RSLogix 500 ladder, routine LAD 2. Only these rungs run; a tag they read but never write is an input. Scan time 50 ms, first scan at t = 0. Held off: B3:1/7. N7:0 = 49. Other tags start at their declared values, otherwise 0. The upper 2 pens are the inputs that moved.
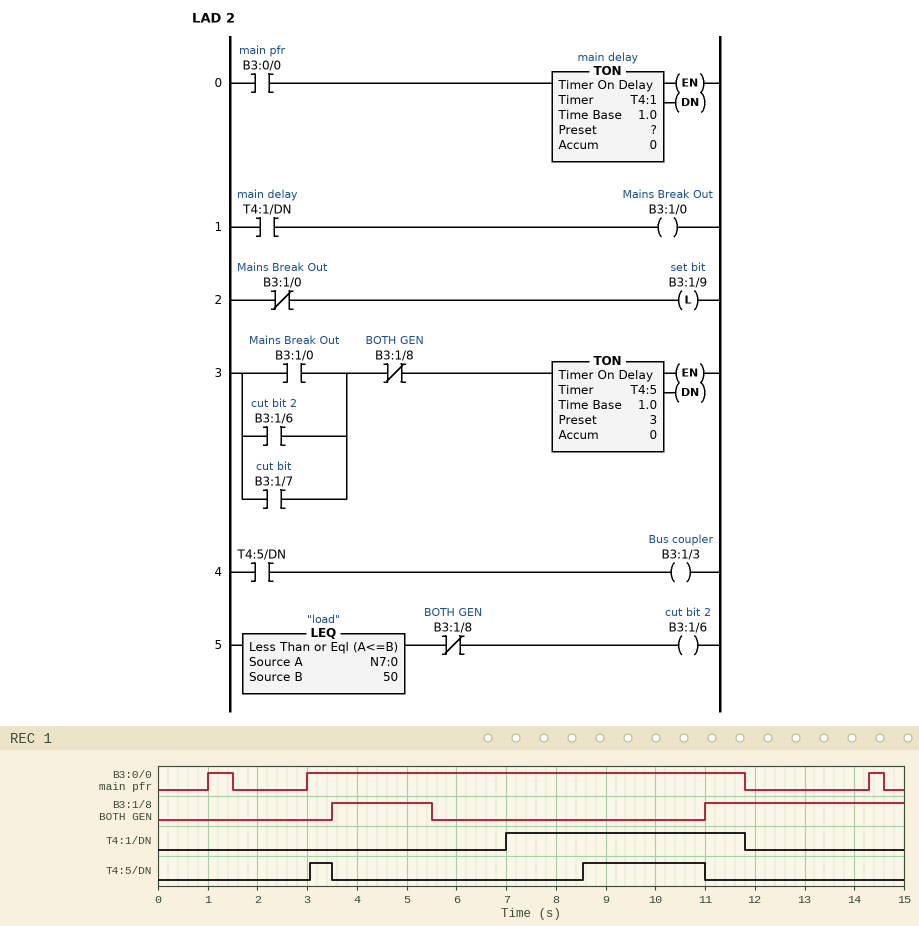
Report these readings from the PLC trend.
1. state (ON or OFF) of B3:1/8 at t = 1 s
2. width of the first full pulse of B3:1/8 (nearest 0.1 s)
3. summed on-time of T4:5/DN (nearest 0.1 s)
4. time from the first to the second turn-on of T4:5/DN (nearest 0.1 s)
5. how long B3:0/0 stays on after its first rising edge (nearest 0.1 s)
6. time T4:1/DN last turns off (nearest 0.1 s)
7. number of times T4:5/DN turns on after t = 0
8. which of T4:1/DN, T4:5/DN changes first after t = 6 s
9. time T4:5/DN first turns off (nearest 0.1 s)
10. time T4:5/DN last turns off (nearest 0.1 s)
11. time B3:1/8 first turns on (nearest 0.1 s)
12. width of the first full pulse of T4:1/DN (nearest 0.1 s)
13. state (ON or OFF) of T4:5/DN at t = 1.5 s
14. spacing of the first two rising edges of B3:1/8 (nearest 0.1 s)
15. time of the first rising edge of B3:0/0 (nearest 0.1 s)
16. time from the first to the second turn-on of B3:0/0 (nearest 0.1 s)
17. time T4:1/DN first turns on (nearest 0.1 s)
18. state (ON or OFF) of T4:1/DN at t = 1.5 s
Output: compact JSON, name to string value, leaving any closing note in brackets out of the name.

{"state (ON or OFF) of B3:1/8 at t = 1 s": "OFF", "width of the first full pulse of B3:1/8": "2.0 s", "summed on-time of T4:5/DN": "2.9 s", "time from the first to the second turn-on of T4:5/DN": "5.5 s", "how long B3:0/0 stays on after its first rising edge": "0.5 s", "time T4:1/DN last turns off": "11.8 s", "number of times T4:5/DN turns on after t = 0": "2", "which of T4:1/DN, T4:5/DN changes first after t = 6 s": "T4:1/DN", "time T4:5/DN first turns off": "3.5 s", "time T4:5/DN last turns off": "11.0 s", "time B3:1/8 first turns on": "3.5 s", "width of the first full pulse of T4:1/DN": "4.8 s", "state (ON or OFF) of T4:5/DN at t = 1.5 s": "OFF", "spacing of the first two rising edges of B3:1/8": "7.5 s", "time of the first rising edge of B3:0/0": "1.0 s", "time from the first to the second turn-on of B3:0/0": "2.0 s", "time T4:1/DN first turns on": "7.0 s", "state (ON or OFF) of T4:1/DN at t = 1.5 s": "OFF"}
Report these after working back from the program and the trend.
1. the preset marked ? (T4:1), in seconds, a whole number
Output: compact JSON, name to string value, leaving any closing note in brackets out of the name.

{"the preset marked ? (T4:1), in seconds, a whole number": "4 s"}
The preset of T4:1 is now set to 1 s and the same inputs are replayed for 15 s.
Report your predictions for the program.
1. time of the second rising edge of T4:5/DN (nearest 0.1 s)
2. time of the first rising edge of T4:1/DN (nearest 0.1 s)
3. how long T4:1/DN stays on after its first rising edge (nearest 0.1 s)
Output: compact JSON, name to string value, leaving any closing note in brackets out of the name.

{"time of the second rising edge of T4:5/DN": "8.5 s", "time of the first rising edge of T4:1/DN": "4.0 s", "how long T4:1/DN stays on after its first rising edge": "7.8 s"}
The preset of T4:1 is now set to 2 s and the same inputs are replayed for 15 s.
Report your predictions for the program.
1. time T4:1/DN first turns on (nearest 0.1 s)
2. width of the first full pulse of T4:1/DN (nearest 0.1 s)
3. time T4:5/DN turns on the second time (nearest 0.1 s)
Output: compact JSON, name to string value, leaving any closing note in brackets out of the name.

{"time T4:1/DN first turns on": "5.0 s", "width of the first full pulse of T4:1/DN": "6.8 s", "time T4:5/DN turns on the second time": "8.5 s"}
